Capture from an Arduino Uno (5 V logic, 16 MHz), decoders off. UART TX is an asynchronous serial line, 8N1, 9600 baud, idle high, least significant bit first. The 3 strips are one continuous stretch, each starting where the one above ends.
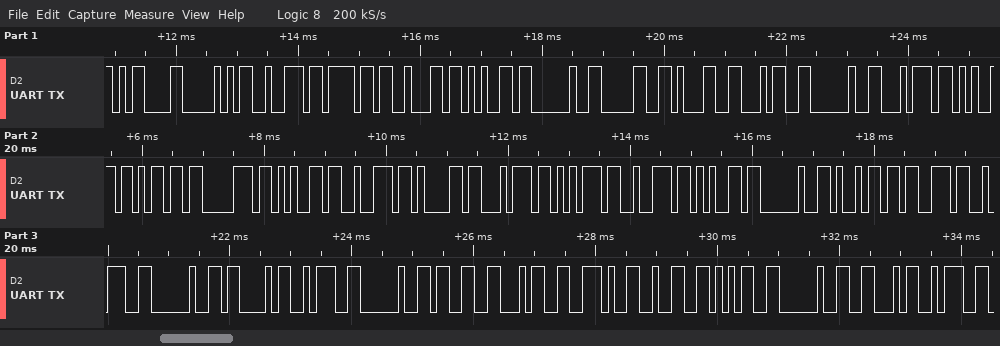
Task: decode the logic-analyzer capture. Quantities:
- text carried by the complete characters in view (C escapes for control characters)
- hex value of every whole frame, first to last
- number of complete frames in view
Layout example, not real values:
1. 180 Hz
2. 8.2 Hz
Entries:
1. "\rProbe 014 temperature is: C: 34.25 F:"
2. 0x0D 0x50 0x72 0x6F 0x62 0x65 0x20 0x30 0x31 0x34 0x20 0x74 0x65 0x6D 0x70 0x65 0x72 0x61 0x74 0x75 0x72 0x65 0x20 0x69 0x73 0x3A 0x20 0x43 0x3A 0x20 0x33 0x34 0x2E 0x32 0x35 0x20 0x46 0x3A
3. 38
